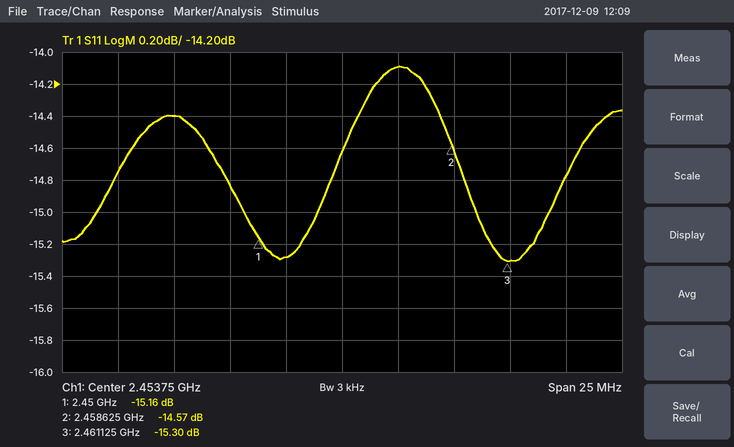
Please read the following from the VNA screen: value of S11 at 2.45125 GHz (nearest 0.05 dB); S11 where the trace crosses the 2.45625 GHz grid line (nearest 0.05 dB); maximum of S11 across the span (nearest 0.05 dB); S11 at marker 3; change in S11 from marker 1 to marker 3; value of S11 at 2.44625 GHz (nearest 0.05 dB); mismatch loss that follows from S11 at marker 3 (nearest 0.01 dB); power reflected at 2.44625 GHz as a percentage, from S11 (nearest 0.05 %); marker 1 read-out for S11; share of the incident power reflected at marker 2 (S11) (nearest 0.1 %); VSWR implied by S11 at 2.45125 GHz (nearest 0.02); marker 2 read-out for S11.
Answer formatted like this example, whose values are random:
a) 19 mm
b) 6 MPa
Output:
a) -15.30 dB
b) -14.10 dB
c) -14.10 dB
d) -15.30 dB
e) -0.14 dB
f) -14.40 dB
g) 0.13 dB
h) 3.65 %
i) -15.16 dB
j) 3.5 %
k) 1.42
l) -14.57 dB
